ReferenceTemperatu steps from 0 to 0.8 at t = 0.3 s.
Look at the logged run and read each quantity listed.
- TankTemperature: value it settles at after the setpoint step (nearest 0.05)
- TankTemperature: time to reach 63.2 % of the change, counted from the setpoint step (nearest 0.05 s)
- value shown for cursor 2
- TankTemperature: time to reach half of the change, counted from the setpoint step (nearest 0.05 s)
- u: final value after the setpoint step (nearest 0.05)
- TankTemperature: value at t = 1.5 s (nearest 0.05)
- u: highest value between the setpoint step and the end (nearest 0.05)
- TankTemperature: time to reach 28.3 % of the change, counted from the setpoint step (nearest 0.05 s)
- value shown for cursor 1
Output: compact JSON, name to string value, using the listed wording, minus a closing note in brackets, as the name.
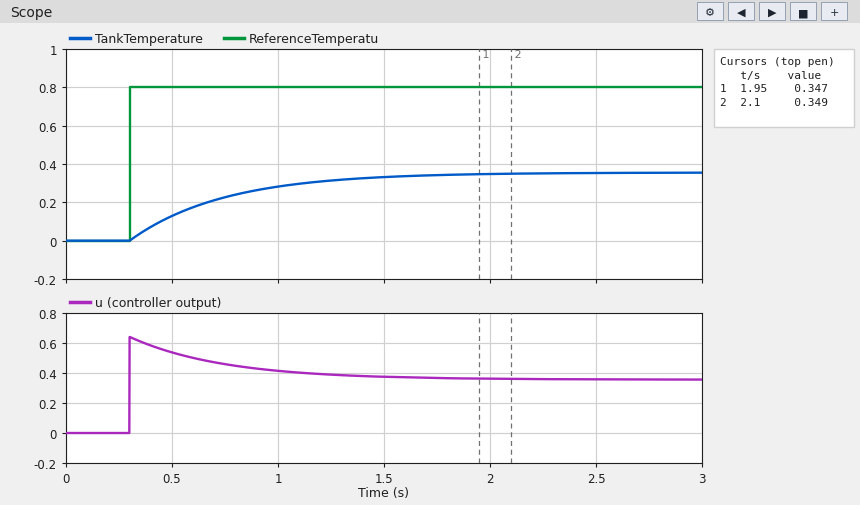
{"TankTemperature: value it settles at after the setpoint step": "0.35", "TankTemperature: time to reach 63.2 % of the change, counted from the setpoint step": "0.45 s", "value shown for cursor 2": "0.349", "TankTemperature: time to reach half of the change, counted from the setpoint step": "0.30 s", "u: final value after the setpoint step": "0.35", "TankTemperature: value at t = 1.5 s": "0.35", "u: highest value between the setpoint step and the end": "0.65", "TankTemperature: time to reach 28.3 % of the change, counted from the setpoint step": "0.15 s", "value shown for cursor 1": "0.347"}
